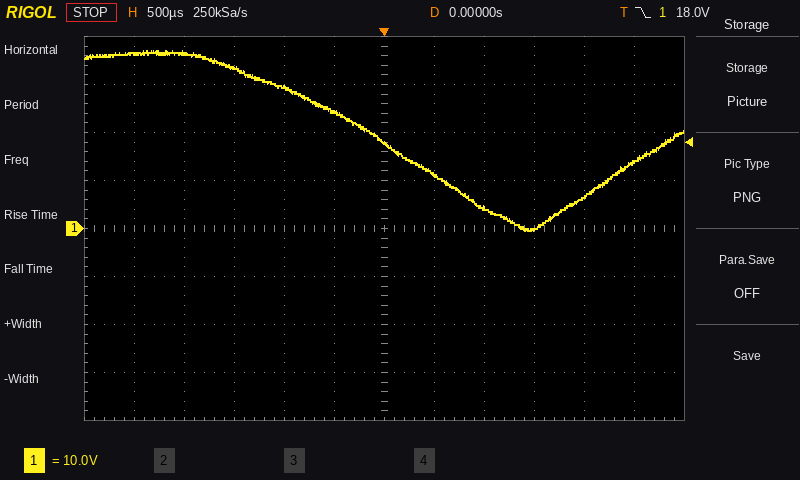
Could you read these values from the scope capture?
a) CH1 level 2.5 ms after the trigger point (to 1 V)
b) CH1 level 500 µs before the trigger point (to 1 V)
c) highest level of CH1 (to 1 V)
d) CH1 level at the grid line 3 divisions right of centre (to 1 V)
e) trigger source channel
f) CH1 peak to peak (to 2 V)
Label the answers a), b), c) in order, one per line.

a) 14 V
b) 24 V
c) 37 V
d) 0 V
e) CH1
f) 38 V
